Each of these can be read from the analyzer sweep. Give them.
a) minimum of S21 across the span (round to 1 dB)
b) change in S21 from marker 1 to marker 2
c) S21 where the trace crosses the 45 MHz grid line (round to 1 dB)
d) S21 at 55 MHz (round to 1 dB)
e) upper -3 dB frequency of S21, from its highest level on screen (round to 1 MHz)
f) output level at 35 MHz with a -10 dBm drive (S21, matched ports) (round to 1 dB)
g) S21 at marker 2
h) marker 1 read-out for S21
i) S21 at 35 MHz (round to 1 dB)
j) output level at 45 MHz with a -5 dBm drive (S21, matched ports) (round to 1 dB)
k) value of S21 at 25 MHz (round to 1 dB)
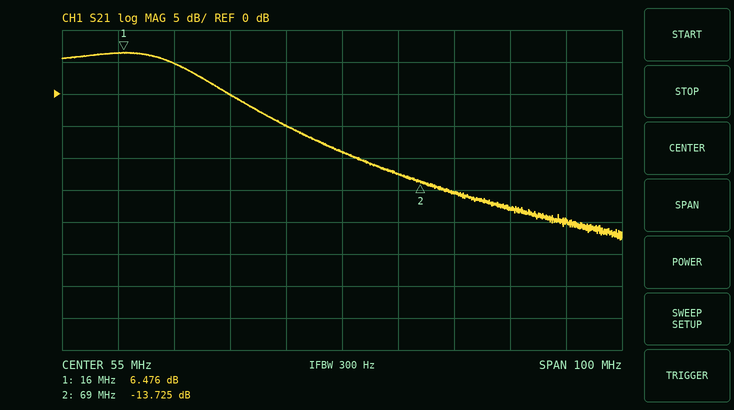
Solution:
-23 dB
-20.201 dB
-5 dB
-9 dB
28 MHz
-10 dBm
-13.725 dB
6.476 dB
0 dB
-10 dBm
5 dB
